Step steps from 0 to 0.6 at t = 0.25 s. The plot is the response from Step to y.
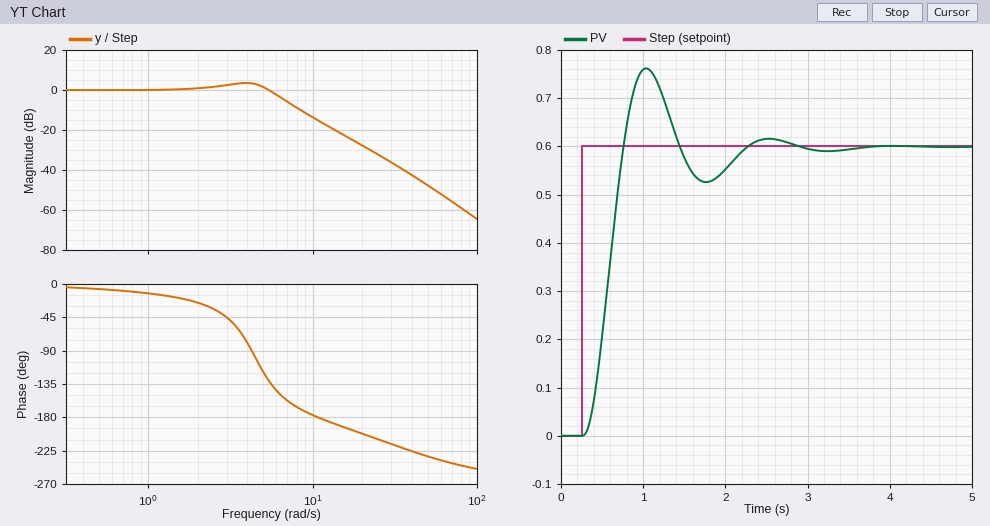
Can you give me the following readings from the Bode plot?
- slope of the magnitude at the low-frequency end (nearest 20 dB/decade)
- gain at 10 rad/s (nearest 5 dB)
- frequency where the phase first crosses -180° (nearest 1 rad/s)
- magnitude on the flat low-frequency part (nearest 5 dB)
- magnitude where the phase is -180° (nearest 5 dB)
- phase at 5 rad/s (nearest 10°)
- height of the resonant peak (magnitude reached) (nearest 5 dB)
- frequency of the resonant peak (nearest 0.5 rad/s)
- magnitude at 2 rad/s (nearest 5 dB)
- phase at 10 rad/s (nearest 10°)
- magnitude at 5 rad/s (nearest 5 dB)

0 dB/decade
-15 dB
11 rad/s
0 dB
-15 dB
-120°
5 dB
4.0 rad/s
0 dB
-180°
0 dB
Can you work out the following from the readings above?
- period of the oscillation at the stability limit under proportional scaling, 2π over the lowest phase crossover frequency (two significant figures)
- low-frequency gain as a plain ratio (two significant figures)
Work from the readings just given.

0.57 s
1.0
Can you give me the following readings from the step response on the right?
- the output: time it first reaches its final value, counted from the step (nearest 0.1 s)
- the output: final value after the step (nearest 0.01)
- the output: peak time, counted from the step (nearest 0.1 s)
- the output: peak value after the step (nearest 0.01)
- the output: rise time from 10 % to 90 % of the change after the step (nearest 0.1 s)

0.5 s
0.60
0.8 s
0.76
0.3 s
